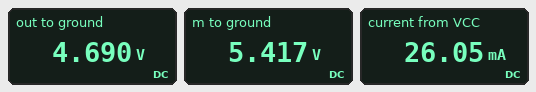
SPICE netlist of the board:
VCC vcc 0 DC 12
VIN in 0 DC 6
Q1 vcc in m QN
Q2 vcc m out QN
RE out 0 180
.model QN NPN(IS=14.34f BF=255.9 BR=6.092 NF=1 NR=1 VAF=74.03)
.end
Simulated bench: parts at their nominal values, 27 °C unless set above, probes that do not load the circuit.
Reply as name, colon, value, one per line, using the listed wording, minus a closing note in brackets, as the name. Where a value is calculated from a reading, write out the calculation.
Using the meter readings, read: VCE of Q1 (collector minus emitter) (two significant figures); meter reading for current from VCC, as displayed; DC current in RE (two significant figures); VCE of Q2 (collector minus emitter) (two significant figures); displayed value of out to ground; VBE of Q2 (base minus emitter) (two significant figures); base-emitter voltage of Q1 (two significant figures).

VCE of Q1 (collector minus emitter): 12 V - 5.417 V = 6.6 V
meter reading for current from VCC, as displayed: 26.05 mA
DC current in RE: (4.69 V) / 180 Ω = 26 mA
VCE of Q2 (collector minus emitter): 12 V - 4.69 V = 7.3 V
displayed value of out to ground: 4.690 V
VBE of Q2 (base minus emitter): 5.417 V - 4.69 V = 730 mV
base-emitter voltage of Q1: 6 V - 5.417 V = 580 mV
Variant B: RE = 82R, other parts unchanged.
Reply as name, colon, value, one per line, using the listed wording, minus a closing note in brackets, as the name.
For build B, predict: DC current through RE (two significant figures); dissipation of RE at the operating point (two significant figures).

DC current through RE: 57 mA
dissipation of RE at the operating point: 260 mW
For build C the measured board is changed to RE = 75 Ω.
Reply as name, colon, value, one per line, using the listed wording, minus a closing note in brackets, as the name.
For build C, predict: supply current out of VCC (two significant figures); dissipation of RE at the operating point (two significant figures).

supply current out of VCC: 62 mA
dissipation of RE at the operating point: 290 mW
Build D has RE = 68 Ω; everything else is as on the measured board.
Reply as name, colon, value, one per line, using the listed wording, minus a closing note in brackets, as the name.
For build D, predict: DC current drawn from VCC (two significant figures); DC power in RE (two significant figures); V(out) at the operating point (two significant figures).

DC current drawn from VCC: 68 mA
DC power in RE: 320 mW
V(out) at the operating point: 4.6 V
